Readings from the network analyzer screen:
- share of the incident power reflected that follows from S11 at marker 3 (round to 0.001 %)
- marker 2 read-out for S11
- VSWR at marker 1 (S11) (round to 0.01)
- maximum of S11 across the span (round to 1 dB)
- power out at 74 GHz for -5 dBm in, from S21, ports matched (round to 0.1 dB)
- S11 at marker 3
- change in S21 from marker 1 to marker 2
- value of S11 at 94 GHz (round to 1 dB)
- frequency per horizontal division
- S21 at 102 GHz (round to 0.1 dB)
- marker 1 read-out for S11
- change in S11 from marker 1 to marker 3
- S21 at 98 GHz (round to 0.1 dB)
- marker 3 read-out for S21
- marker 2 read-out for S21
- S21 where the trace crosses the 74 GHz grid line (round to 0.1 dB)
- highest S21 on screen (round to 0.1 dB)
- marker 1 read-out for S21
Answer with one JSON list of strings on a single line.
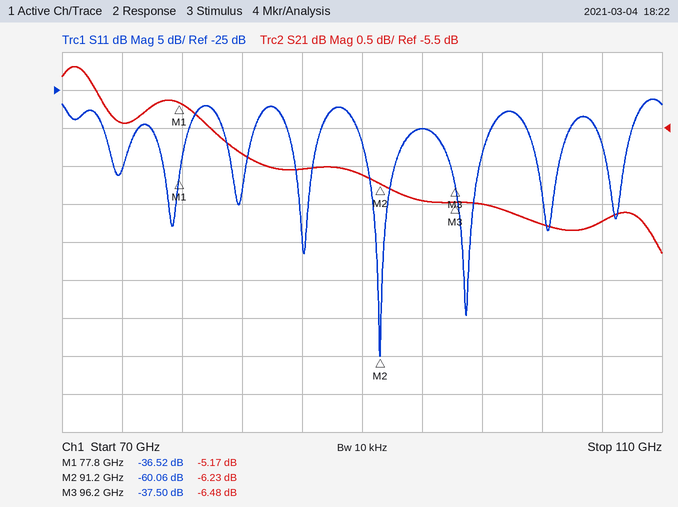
["0.018 %", "-60.06 dB", "1.03", "-26 dB", "-10.4 dBm", "-37.50 dB", "-1.06 dB", "-30 dB", "4 GHz", "-6.8 dB", "-36.52 dB", "-0.98 dB", "-6.5 dB", "-6.48 dB", "-6.23 dB", "-5.4 dB", "-4.7 dB", "-5.17 dB"]
